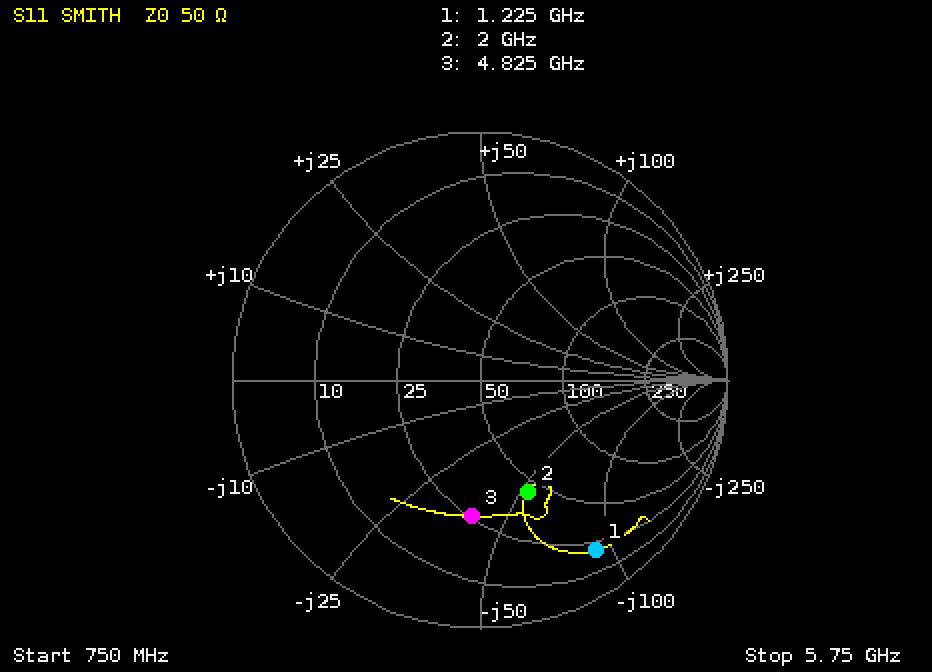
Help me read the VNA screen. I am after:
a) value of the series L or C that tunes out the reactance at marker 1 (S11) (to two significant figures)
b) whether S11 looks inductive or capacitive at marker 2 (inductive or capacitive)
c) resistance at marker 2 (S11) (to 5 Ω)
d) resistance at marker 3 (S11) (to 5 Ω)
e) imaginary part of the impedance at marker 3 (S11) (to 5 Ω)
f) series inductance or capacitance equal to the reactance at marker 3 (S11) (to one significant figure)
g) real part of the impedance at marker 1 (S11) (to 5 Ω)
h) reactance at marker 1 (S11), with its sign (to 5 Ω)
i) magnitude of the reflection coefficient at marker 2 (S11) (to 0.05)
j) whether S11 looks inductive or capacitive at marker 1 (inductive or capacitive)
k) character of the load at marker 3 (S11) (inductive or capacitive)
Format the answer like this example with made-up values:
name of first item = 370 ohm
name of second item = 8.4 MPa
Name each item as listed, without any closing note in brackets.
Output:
value of the series L or C that tunes out the reactance at marker 1 (S11) = 12 nH
whether S11 looks inductive or capacitive at marker 2 = capacitive
resistance at marker 2 (S11) = 45 Ω
resistance at marker 3 (S11) = 25 Ω
imaginary part of the impedance at marker 3 (S11) = -40 Ω
series inductance or capacitance equal to the reactance at marker 3 (S11) = 800 fF
real part of the impedance at marker 1 (S11) = 20 Ω
reactance at marker 1 (S11), with its sign = -90 Ω
magnitude of the reflection coefficient at marker 2 (S11) = 0.50
whether S11 looks inductive or capacitive at marker 1 = capacitive
character of the load at marker 3 (S11) = capacitive
